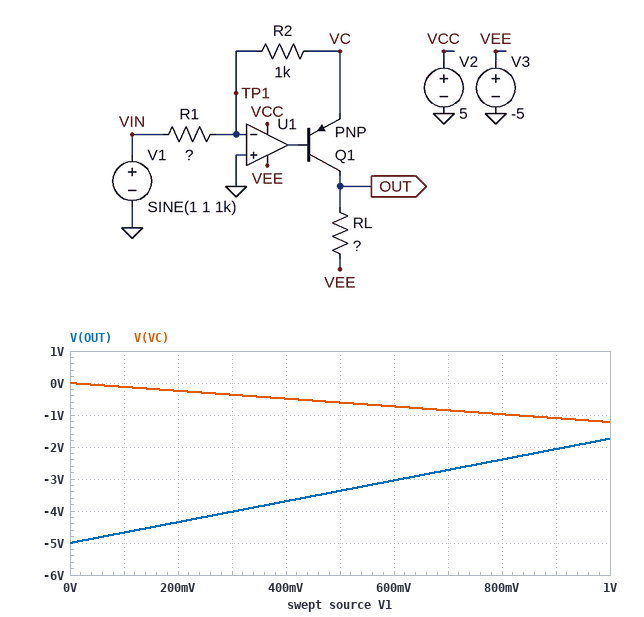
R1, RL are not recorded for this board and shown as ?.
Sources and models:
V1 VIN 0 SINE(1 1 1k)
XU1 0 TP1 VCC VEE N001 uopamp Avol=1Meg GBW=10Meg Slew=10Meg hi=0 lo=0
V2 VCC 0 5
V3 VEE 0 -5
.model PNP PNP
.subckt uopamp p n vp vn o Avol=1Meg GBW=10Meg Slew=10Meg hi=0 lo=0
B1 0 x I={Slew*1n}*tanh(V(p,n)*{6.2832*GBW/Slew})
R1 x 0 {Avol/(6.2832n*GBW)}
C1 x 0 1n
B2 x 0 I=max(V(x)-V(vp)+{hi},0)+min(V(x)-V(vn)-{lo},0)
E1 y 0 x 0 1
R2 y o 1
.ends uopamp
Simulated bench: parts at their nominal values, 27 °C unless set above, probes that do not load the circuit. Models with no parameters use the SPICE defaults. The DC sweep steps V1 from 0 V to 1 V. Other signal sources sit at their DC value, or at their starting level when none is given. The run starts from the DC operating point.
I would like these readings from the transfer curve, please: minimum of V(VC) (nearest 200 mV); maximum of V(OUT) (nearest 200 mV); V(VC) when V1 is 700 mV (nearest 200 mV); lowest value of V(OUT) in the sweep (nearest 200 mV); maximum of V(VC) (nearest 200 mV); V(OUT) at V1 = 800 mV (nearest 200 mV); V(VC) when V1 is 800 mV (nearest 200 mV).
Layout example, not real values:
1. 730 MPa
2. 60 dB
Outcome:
1. -1.2 V
2. -1.8 V
3. -800 mV
4. -5.0 V
5. 0 V
6. -2.4 V
7. -1.0 V
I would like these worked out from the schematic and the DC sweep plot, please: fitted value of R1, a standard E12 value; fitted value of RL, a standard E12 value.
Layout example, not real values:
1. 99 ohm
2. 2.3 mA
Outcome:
1. 820 Ω
2. 2.7 kΩ
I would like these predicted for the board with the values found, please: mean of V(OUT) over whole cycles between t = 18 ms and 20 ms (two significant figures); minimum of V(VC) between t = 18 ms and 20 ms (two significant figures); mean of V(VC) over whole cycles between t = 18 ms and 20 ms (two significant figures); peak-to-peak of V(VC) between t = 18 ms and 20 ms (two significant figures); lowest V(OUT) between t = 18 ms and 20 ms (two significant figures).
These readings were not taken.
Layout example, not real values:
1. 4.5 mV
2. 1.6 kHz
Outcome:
1. -2.9 V
2. -2.4 V
3. -1.2 V
4. 2.4 V
5. -5.0 V
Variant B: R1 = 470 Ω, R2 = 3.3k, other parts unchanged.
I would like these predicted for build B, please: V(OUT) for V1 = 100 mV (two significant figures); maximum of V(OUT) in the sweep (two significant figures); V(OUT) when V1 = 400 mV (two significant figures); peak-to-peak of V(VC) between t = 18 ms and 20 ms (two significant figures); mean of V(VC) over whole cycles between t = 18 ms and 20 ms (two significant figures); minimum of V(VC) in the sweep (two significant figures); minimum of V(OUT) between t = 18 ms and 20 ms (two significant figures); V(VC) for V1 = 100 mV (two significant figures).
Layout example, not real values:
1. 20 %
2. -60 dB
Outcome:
1. -4.4 V
2. -2.8 V
3. -2.9 V
4. 4.2 V
5. -3.2 V
6. -4.2 V
7. -5.0 V
8. -700 mV
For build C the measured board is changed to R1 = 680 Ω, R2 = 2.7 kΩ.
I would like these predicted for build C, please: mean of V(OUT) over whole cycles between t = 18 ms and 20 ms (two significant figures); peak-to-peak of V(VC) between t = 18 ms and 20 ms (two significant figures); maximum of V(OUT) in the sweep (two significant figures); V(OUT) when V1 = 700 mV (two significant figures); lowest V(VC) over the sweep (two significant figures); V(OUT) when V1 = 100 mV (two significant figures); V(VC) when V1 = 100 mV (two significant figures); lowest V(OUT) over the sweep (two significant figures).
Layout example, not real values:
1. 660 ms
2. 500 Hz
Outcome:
1. -4.1 V
2. 4.2 V
3. -2.6 V
4. -2.8 V
5. -4.0 V
6. -4.6 V
7. -400 mV
8. -5.0 V
